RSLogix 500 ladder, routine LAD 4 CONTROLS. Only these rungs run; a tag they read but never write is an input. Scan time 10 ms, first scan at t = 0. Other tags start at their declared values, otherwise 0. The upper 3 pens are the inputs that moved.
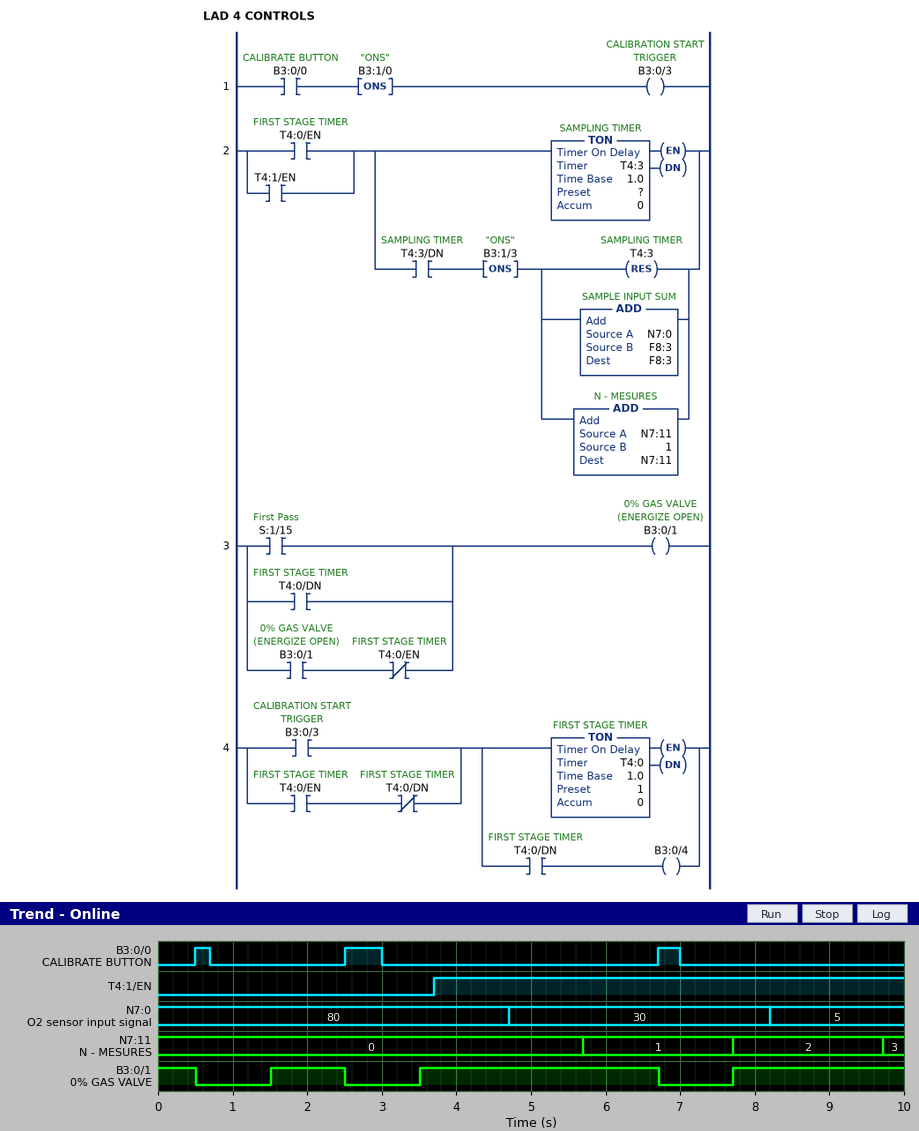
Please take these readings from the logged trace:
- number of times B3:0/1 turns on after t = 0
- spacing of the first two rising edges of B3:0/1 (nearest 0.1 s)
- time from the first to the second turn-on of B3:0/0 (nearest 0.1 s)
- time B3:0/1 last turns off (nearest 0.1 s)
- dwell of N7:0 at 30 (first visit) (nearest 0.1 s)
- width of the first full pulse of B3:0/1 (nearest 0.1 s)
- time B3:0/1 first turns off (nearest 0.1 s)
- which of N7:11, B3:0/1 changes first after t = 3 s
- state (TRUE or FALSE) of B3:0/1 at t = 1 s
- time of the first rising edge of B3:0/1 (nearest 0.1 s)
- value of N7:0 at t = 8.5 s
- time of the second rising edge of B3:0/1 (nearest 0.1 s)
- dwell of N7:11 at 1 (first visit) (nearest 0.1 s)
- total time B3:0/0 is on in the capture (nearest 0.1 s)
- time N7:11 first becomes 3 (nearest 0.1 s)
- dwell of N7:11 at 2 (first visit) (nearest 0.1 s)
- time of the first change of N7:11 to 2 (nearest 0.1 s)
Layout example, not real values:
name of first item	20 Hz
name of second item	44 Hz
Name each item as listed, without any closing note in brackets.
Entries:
number of times B3:0/1 turns on after t = 0	3
spacing of the first two rising edges of B3:0/1	2.0 s
time from the first to the second turn-on of B3:0/0	2.0 s
time B3:0/1 last turns off	6.7 s
dwell of N7:0 at 30 (first visit)	3.5 s
width of the first full pulse of B3:0/1	1.0 s
time B3:0/1 first turns off	0.5 s
which of N7:11, B3:0/1 changes first after t = 3 s	B3:0/1
state (TRUE or FALSE) of B3:0/1 at t = 1 s	FALSE
time of the first rising edge of B3:0/1	1.5 s
value of N7:0 at t = 8.5 s	5
time of the second rising edge of B3:0/1	3.5 s
dwell of N7:11 at 1 (first visit)	2.0 s
total time B3:0/0 is on in the capture	1.0 s
time N7:11 first becomes 3	9.7 s
dwell of N7:11 at 2 (first visit)	2.0 s
time of the first change of N7:11 to 2	7.7 s
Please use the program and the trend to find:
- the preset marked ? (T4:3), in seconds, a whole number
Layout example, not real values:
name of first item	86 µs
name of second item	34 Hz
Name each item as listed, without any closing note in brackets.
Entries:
the preset marked ? (T4:3), in seconds, a whole number	2 s
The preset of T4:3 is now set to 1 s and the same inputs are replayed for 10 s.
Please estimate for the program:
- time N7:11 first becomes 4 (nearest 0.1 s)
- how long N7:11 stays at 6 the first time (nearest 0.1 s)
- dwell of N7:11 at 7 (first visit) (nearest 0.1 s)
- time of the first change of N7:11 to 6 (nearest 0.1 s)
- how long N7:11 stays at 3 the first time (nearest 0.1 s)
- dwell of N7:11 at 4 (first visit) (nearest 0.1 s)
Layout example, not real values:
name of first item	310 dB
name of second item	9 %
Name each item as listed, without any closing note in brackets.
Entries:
time N7:11 first becomes 4	5.7 s
how long N7:11 stays at 6 the first time	1.0 s
dwell of N7:11 at 7 (first visit)	1.0 s
time of the first change of N7:11 to 6	7.7 s
how long N7:11 stays at 3 the first time	1.0 s
dwell of N7:11 at 4 (first visit)	1.0 s
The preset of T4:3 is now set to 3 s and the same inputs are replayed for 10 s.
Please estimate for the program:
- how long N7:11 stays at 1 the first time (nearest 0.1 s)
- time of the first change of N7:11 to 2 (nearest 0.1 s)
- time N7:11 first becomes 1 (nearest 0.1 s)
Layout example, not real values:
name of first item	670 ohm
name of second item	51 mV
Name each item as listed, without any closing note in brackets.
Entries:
how long N7:11 stays at 1 the first time	3.0 s
time of the first change of N7:11 to 2	9.7 s
time N7:11 first becomes 1	6.7 s
